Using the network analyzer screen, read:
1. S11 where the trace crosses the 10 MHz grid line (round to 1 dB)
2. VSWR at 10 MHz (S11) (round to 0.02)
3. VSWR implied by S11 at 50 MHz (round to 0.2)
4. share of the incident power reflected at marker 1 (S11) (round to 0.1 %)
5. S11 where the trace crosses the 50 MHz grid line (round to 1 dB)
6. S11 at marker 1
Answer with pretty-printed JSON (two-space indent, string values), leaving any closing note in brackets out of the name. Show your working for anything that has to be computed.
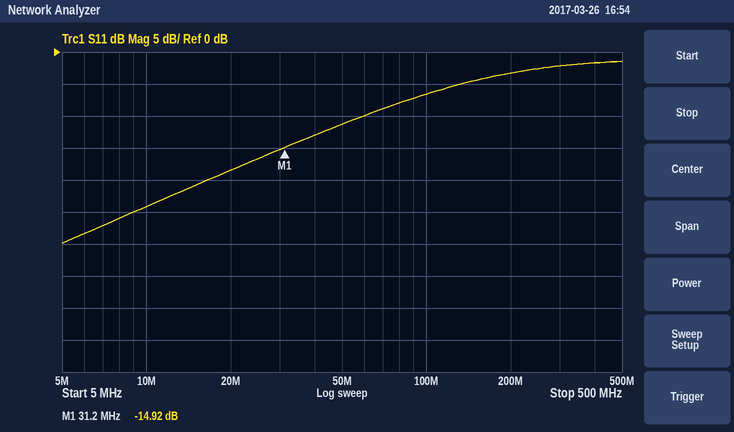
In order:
{
  "S11 where the trace crosses the 10 MHz grid line": "-24 dB",
  "VSWR at 10 MHz (S11)": "|Γ| = 10^(-24/20) = 0.0631; VSWR = (1 + 0.0631)/(1 − 0.0631) ≈ 1.13, so 1.14 to the nearest 0.02",
  "VSWR implied by S11 at 50 MHz": "|Γ| = 10^(-11/20) = 0.2818; VSWR = (1 + 0.2818)/(1 − 0.2818) ≈ 1.8",
  "share of the incident power reflected at marker 1 (S11)": "10^(-14.92/10) ≈ 3.2 %",
  "S11 where the trace crosses the 50 MHz grid line": "-11 dB",
  "S11 at marker 1": "-14.92 dB"
}
